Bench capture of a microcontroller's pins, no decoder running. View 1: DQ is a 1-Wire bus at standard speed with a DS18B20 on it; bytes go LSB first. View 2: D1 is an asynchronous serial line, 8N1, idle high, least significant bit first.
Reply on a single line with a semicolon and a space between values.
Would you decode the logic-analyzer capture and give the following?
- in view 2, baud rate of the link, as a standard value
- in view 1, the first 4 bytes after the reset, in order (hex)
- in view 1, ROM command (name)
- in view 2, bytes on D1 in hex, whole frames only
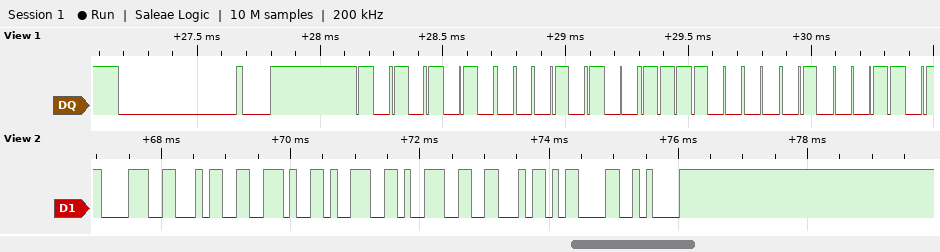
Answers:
9600 baud; 55 28 0F 62; Match ROM; 38 34 2E 39 39 46 0D 0A
